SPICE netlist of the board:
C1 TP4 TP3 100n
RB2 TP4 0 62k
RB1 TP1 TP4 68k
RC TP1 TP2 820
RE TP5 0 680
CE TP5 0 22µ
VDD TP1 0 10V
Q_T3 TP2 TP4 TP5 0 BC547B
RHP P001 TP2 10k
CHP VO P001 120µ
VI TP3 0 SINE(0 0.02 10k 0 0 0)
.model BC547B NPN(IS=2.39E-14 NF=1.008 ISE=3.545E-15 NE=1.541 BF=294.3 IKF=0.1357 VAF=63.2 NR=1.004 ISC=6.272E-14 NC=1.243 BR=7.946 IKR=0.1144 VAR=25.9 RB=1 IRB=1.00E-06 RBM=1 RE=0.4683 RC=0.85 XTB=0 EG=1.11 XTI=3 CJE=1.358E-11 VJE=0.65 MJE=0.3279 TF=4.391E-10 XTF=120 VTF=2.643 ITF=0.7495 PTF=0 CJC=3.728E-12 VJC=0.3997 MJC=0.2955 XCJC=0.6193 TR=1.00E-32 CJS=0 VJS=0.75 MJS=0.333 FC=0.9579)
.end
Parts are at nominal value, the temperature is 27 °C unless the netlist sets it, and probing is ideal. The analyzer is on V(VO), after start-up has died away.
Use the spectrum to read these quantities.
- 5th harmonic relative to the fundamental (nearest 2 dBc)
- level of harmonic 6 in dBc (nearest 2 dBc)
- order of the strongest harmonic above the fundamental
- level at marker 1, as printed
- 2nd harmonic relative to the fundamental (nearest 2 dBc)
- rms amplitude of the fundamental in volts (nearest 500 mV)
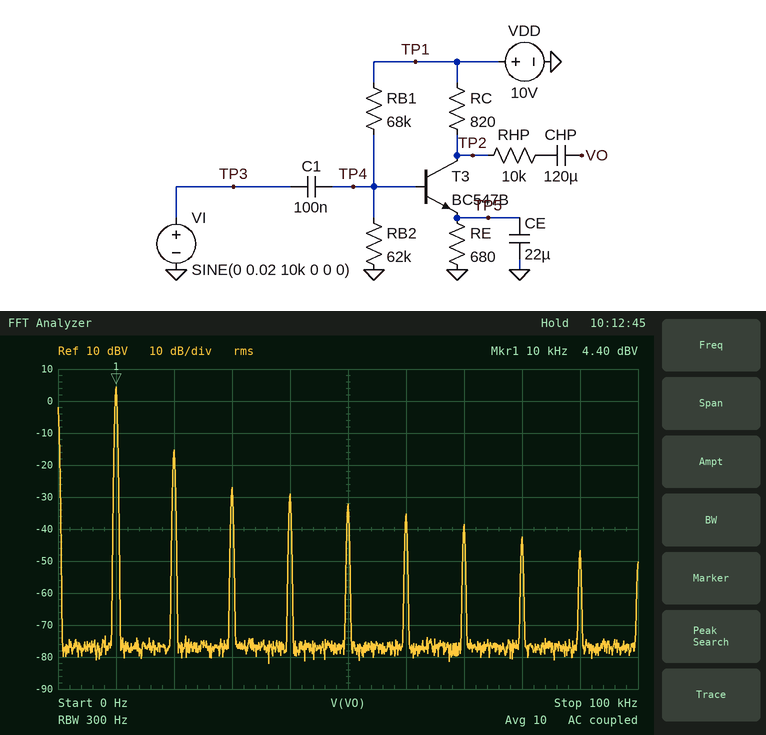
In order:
-36 dBc
-40 dBc
2
4.40 dBV
-20 dBc
1.5 V
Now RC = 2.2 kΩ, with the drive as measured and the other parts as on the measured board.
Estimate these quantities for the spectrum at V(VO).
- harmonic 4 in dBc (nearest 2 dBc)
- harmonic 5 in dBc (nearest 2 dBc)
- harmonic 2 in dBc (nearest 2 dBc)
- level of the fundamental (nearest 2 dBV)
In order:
-22 dBc
-30 dBc
-8 dBc
2 dBV
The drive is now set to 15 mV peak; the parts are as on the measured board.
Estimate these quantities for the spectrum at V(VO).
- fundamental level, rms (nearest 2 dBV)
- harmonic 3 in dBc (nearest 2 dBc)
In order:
2 dBV
-48 dBc
